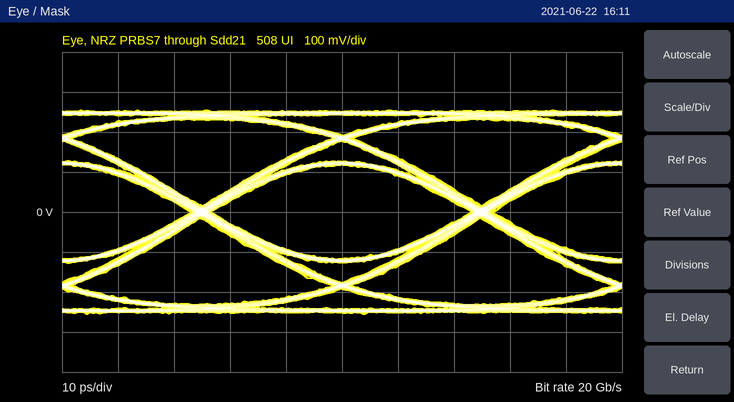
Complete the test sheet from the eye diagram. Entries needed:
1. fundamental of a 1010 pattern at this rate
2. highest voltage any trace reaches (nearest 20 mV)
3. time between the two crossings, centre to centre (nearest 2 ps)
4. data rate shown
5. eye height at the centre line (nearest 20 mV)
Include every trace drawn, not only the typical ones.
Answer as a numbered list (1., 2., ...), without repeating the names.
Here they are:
1. 10 GHz
2. 260 mV
3. 50 ps
4. 20 Gb/s
5. 240 mV
